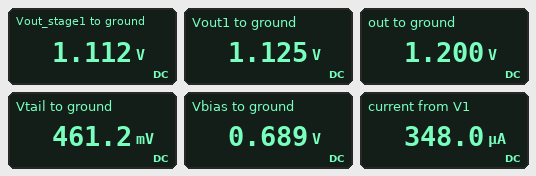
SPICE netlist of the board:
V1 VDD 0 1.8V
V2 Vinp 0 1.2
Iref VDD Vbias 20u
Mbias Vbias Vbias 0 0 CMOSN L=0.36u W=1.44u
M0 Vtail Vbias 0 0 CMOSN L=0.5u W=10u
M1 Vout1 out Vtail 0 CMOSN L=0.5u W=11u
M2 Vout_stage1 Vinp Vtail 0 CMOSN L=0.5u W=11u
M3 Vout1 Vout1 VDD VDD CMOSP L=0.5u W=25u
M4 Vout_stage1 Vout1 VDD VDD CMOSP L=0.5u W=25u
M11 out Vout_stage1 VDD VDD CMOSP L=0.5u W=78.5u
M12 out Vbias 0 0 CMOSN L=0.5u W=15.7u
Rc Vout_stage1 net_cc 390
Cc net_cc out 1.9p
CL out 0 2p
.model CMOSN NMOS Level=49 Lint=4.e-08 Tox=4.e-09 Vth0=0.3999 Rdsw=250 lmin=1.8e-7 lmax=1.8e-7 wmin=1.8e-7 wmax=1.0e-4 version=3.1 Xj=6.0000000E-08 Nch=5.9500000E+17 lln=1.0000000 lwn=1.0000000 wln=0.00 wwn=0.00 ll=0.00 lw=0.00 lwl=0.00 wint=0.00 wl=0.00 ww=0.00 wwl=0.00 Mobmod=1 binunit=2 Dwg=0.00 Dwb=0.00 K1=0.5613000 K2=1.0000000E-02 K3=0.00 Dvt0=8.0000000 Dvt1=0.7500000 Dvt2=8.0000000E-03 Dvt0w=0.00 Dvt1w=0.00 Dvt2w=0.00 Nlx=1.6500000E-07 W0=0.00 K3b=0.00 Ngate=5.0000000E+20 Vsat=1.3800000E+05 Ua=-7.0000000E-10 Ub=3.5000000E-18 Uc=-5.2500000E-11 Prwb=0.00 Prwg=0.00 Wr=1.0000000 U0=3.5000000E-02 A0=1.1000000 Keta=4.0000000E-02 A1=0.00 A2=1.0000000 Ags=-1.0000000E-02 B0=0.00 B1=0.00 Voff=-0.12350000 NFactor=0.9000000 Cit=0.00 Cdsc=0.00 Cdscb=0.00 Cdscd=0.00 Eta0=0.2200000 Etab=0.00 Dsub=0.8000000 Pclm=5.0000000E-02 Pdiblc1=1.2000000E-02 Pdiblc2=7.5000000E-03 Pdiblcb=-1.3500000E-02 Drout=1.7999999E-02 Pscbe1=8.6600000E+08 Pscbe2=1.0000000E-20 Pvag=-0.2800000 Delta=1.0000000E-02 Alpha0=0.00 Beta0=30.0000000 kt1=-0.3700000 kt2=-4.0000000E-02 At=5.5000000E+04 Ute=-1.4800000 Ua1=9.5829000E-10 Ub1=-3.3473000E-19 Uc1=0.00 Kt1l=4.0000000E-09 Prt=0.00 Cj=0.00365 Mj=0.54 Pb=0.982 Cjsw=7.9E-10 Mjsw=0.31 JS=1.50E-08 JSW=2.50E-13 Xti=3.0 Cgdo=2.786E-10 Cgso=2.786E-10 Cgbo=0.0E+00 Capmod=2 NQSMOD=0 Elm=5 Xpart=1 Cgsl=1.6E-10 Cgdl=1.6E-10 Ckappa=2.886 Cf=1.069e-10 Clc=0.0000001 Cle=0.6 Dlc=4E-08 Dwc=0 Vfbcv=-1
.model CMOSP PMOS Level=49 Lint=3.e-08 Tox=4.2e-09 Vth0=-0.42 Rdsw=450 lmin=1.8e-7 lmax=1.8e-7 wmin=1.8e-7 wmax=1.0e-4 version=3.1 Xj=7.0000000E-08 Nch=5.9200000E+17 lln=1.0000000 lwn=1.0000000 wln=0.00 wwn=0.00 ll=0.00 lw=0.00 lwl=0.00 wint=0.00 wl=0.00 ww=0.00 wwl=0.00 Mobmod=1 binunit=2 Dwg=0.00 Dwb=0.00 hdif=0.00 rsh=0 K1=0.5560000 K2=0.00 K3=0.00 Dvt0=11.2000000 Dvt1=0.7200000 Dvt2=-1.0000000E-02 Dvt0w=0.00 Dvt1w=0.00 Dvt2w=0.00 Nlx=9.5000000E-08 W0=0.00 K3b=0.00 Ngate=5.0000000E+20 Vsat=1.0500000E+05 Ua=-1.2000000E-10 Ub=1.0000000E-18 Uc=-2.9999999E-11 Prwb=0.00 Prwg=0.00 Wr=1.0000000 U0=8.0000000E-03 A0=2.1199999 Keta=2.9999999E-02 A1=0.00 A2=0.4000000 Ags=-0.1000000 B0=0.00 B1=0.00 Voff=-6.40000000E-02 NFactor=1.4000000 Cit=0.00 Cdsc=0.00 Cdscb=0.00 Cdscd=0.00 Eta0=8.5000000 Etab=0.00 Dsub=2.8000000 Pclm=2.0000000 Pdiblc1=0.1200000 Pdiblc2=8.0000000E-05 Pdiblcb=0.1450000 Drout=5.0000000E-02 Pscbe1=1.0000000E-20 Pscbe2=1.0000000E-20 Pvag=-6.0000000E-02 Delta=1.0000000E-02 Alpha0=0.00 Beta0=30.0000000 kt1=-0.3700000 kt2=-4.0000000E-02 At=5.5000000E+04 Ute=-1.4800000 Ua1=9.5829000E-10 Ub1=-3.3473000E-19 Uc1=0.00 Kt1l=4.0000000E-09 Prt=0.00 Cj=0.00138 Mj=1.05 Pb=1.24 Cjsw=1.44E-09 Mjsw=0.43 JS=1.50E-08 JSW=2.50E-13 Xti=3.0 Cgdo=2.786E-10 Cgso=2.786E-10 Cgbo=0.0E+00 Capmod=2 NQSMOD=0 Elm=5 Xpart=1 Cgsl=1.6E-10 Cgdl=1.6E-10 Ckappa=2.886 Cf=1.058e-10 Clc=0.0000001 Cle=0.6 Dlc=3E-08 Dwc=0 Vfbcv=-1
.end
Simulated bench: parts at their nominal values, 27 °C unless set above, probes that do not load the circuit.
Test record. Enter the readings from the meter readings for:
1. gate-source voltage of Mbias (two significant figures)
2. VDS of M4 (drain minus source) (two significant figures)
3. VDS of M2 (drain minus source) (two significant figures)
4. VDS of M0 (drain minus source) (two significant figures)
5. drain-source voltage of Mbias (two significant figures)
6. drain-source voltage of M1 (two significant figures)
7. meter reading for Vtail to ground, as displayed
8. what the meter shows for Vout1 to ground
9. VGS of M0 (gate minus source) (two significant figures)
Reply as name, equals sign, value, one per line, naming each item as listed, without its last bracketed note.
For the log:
gate-source voltage of Mbias = 690 mV
VDS of M4 (drain minus source) = -690 mV
VDS of M2 (drain minus source) = 650 mV
VDS of M0 (drain minus source) = 460 mV
drain-source voltage of Mbias = 690 mV
drain-source voltage of M1 = 660 mV
meter reading for Vtail to ground, as displayed = 461.2 mV
what the meter shows for Vout1 to ground = 1.125 V
VGS of M0 (gate minus source) = 690 mV
